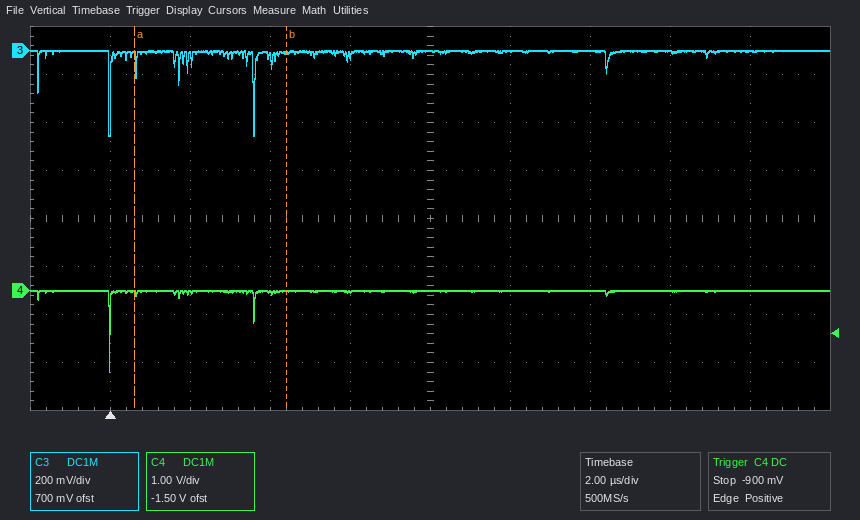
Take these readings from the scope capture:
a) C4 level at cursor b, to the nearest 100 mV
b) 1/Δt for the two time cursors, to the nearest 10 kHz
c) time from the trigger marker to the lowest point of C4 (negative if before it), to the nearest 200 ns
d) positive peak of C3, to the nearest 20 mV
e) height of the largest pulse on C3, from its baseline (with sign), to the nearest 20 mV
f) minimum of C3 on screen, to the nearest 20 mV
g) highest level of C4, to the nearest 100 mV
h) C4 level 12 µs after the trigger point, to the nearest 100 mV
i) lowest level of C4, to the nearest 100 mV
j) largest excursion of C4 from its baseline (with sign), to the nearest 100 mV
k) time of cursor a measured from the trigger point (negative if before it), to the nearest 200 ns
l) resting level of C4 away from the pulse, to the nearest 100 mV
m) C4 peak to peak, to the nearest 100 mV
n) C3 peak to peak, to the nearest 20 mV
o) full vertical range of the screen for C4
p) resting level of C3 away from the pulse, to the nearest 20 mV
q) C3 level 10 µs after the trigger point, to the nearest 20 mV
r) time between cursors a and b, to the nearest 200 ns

0.0 V
260 kHz
0.0 µs
0 mV
-360 mV
-360 mV
0.0 V
0.0 V
-1.7 V
-1.7 V
+600 ns
0.0 V
1.7 V
360 mV
8 V
0 mV
0 mV
3.8 µs
